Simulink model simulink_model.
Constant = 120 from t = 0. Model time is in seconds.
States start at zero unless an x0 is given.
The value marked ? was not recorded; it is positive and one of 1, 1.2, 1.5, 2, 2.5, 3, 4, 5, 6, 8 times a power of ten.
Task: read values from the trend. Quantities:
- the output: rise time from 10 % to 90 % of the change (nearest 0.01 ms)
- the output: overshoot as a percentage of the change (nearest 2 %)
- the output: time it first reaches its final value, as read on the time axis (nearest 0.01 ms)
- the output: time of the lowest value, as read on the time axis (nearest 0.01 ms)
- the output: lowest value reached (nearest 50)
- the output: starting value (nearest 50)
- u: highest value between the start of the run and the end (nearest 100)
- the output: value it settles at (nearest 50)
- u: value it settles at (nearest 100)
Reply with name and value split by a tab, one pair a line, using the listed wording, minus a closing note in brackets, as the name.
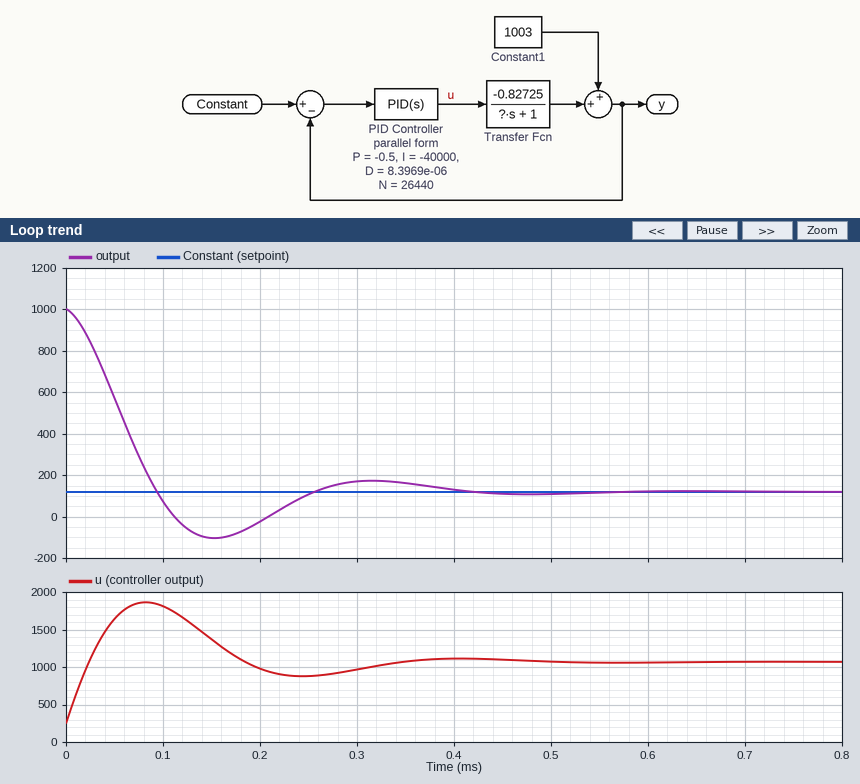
the output: rise time from 10 % to 90 % of the change	0.07 ms
the output: overshoot as a percentage of the change	26 %
the output: time it first reaches its final value, as read on the time axis	0.09 ms
the output: time of the lowest value, as read on the time axis	0.15 ms
the output: lowest value reached	-100
the output: starting value	1000
u: highest value between the start of the run and the end	1900
the output: value it settles at	100
u: value it settles at	1100
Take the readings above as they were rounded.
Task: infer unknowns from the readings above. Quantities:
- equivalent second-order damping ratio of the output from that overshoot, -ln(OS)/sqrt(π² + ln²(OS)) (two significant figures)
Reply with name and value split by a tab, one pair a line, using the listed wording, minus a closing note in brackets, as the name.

equivalent second-order damping ratio of the output from that overshoot, -ln(OS)/sqrt(π² + ln²(OS))	0.39
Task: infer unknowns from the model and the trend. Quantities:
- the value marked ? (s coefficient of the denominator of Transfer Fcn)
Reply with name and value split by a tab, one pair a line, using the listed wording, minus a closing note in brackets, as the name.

the value marked ?	8e-05
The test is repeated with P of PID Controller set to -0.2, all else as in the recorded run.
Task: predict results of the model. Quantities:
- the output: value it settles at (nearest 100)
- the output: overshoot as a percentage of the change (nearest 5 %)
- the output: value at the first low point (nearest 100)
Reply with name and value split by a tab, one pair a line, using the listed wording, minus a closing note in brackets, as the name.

the output: value it settles at	100
the output: overshoot as a percentage of the change	35 %
the output: value at the first low point	-200
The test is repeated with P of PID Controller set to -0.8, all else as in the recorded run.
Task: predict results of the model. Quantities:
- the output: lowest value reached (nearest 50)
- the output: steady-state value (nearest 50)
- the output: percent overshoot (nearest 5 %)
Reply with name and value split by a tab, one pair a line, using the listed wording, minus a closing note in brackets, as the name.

the output: lowest value reached	-50
the output: steady-state value	100
the output: percent overshoot	20 %
